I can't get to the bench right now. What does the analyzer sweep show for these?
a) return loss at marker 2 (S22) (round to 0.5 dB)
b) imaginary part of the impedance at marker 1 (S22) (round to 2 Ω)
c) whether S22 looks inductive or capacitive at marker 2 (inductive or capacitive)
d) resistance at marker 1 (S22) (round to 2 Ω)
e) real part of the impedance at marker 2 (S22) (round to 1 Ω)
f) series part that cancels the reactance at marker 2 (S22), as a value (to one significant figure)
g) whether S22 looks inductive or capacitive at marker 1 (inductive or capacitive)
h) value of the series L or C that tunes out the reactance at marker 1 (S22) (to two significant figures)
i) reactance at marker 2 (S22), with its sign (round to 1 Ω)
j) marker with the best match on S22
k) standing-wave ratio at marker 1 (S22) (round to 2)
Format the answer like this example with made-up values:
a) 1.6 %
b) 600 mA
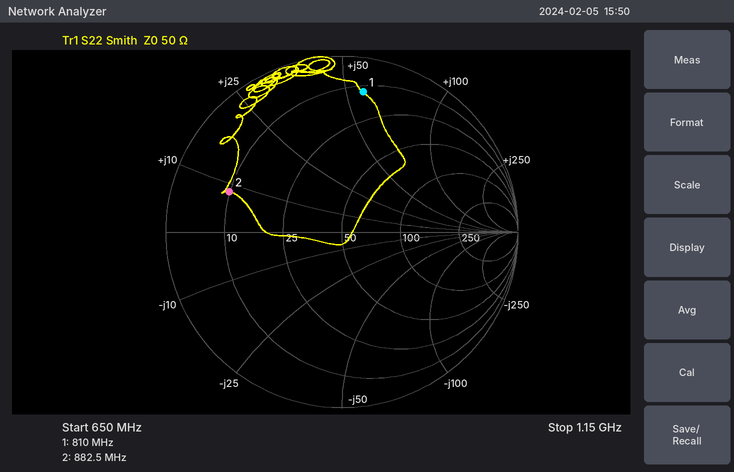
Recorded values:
a) 3.5 dB
b) +56 Ω
c) inductive
d) 12 Ω
e) 10 Ω
f) 20 pF
g) inductive
h) 3.5 pF
i) +8 Ω
j) marker 2
k) 10
